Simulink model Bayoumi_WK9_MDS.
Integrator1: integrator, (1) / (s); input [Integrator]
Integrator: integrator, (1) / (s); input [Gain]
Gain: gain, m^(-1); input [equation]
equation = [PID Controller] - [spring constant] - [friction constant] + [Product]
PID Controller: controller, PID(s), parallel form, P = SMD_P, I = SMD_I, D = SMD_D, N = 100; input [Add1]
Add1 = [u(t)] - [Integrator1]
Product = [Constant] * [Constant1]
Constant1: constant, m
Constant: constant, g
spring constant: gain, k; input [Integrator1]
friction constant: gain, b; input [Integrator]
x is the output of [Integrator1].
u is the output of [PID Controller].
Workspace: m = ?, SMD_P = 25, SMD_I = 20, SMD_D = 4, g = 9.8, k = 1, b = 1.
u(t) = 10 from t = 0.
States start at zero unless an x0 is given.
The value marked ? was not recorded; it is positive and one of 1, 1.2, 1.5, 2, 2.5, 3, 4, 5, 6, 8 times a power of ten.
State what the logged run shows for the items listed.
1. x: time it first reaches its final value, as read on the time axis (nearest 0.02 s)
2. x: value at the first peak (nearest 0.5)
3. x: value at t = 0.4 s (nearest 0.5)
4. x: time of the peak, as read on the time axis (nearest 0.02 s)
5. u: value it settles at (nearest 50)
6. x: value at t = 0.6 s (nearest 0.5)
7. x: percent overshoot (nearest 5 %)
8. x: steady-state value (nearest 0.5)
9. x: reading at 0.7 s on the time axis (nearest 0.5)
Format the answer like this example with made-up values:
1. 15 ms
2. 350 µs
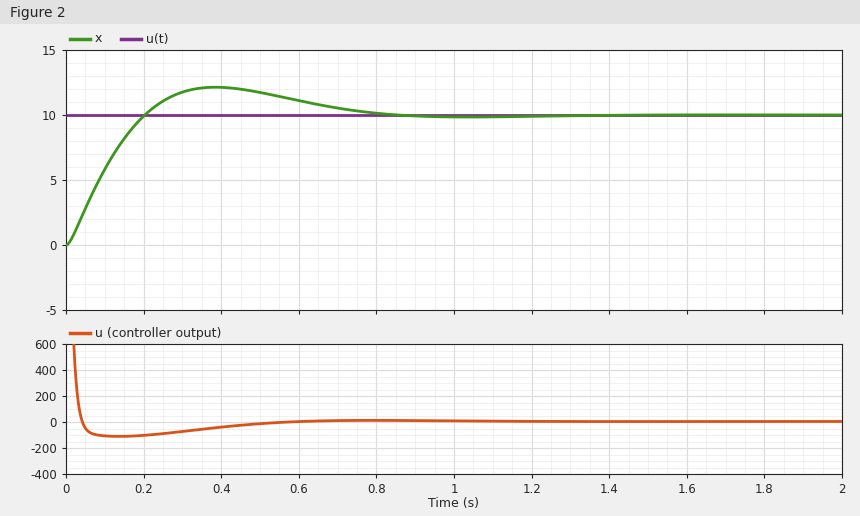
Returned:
1. 0.20 s
2. 12.0
3. 12.0
4. 0.38 s
5. 0
6. 11.0
7. 20 %
8. 10.0
9. 10.5
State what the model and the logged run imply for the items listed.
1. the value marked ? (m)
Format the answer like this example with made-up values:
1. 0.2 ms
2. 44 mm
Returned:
1. 0.6
